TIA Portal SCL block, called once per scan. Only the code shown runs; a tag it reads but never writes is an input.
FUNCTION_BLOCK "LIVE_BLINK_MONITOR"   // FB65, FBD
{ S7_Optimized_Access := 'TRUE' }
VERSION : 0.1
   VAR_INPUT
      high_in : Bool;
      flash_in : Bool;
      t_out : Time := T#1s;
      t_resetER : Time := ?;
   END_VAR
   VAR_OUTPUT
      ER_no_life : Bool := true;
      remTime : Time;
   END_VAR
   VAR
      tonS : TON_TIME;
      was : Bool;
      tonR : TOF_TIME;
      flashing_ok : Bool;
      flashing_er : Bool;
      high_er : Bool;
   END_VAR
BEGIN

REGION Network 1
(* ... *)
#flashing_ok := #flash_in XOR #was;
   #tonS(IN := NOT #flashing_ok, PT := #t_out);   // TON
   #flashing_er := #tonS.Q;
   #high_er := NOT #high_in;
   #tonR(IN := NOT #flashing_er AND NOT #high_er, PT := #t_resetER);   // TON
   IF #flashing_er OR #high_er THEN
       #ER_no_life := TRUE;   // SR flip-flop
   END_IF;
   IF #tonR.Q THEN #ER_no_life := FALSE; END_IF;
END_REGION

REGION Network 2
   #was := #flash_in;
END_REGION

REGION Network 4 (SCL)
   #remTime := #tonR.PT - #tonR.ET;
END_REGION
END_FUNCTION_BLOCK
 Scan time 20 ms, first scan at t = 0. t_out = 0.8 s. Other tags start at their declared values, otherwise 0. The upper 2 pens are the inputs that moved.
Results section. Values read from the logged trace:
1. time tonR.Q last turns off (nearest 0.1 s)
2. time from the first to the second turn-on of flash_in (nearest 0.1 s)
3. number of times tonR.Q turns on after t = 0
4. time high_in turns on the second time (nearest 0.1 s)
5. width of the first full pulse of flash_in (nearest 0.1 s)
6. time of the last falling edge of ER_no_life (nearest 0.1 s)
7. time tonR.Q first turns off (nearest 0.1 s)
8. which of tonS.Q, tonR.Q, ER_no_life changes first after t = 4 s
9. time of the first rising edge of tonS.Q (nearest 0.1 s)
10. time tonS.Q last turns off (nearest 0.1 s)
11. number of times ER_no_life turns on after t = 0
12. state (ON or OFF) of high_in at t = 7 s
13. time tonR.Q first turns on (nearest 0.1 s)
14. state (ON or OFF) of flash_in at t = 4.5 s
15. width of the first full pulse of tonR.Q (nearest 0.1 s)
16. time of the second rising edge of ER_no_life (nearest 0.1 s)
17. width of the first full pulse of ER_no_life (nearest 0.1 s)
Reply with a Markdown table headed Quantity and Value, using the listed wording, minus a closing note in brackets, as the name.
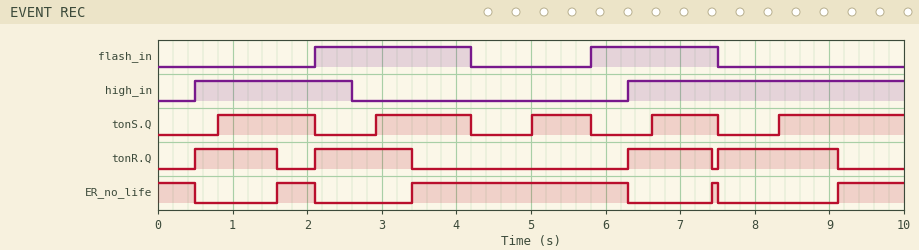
| Quantity | Value |
|---|---|
| time tonR.Q last turns off | 9.1 s |
| time from the first to the second turn-on of flash_in | 3.7 s |
| number of times tonR.Q turns on after t = 0 | 4 |
| time high_in turns on the second time | 6.3 s |
| width of the first full pulse of flash_in | 2.1 s |
| time of the last falling edge of ER_no_life | 7.5 s |
| time tonR.Q first turns off | 1.6 s |
| which of tonS.Q, tonR.Q, ER_no_life changes first after t = 4 s | tonS.Q |
| time of the first rising edge of tonS.Q | 0.8 s |
| time tonS.Q last turns off | 7.5 s |
| number of times ER_no_life turns on after t = 0 | 4 |
| state (ON or OFF) of high_in at t = 7 s | ON |
| time tonR.Q first turns on | 0.5 s |
| state (ON or OFF) of flash_in at t = 4.5 s | OFF |
| width of the first full pulse of tonR.Q | 1.1 s |
| time of the second rising edge of ER_no_life | 3.4 s |
| width of the first full pulse of ER_no_life | 0.5 s |
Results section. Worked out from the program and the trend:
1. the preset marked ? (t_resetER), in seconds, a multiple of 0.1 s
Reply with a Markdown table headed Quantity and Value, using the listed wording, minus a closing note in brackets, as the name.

| Quantity | Value |
|---|---|
| the preset marked ? (t_resetER), in seconds, a multiple of 0.1 s | 0.8 s |
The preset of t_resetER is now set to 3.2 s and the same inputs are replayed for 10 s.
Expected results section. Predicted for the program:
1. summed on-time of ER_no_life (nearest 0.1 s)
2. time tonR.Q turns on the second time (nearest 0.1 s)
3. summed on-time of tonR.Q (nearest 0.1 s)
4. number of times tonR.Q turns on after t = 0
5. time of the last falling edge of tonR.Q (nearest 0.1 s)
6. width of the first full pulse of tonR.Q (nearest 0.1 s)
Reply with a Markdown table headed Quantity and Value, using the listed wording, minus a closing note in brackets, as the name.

| Quantity | Value |
|---|---|
| summed on-time of ER_no_life | 1.0 s |
| time tonR.Q turns on the second time | 6.3 s |
| summed on-time of tonR.Q | 9.0 s |
| number of times tonR.Q turns on after t = 0 | 2 |
| time of the last falling edge of tonR.Q | 5.8 s |
| width of the first full pulse of tonR.Q | 5.3 s |
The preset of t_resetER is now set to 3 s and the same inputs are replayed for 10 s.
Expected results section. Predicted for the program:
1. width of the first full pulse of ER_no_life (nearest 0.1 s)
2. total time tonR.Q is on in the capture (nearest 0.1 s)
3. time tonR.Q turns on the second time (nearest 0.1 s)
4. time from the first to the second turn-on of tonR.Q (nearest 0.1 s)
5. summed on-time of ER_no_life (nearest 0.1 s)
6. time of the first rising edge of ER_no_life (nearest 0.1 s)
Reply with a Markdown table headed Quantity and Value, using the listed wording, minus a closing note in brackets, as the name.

| Quantity | Value |
|---|---|
| width of the first full pulse of ER_no_life | 0.7 s |
| total time tonR.Q is on in the capture | 8.8 s |
| time tonR.Q turns on the second time | 6.3 s |
| time from the first to the second turn-on of tonR.Q | 5.8 s |
| summed on-time of ER_no_life | 1.2 s |
| time of the first rising edge of ER_no_life | 5.6 s |
